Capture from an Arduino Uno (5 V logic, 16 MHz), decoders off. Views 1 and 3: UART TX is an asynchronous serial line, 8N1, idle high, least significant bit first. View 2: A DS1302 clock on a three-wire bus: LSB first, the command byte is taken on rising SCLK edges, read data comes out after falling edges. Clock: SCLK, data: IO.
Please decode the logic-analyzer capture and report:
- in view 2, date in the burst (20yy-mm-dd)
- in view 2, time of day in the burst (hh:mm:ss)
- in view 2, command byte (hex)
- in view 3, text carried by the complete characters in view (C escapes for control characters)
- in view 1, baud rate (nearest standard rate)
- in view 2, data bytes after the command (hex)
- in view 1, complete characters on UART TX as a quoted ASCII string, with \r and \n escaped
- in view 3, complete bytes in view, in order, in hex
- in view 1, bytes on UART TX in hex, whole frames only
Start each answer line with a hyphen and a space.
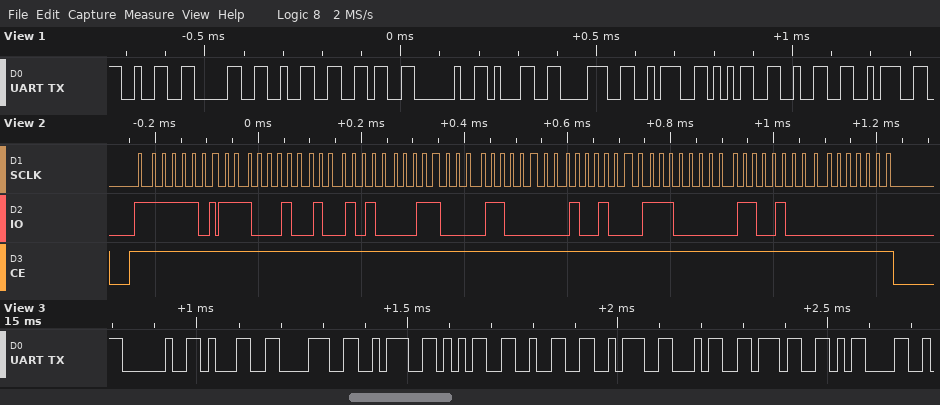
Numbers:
- 2026-12-06
- 18:52:47
- 0xBF
- " 18:52:47\r"
- 57600 baud
- 47 52 18 06 12 07 26 00
- "2026 18:52:"
- 20 31 38 3A 35 32 3A 34 37 0D
- 0x32 0x30 0x32 0x36 0x20 0x31 0x38 0x3A 0x35 0x32 0x3A
